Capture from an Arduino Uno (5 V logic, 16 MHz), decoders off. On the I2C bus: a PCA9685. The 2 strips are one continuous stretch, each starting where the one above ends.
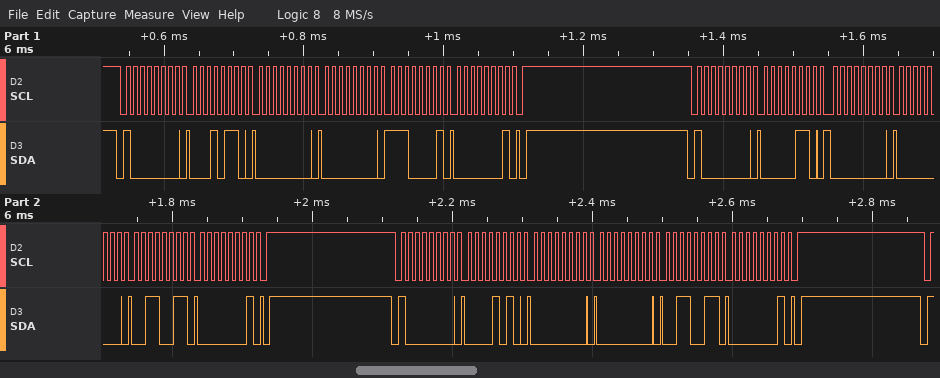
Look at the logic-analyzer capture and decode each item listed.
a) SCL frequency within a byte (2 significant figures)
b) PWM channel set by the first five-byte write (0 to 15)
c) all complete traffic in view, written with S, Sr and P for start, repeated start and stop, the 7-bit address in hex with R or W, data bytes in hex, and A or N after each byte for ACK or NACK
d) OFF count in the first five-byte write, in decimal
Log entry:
100 kHz
4
S 40W A 16 A 00 A 00 A E1 A 01 A P S 40W A 06 A 00 A 00 A 33 A 01 A P S 40W A 0A A 00 A 00 A 33 A 01 A P
481
